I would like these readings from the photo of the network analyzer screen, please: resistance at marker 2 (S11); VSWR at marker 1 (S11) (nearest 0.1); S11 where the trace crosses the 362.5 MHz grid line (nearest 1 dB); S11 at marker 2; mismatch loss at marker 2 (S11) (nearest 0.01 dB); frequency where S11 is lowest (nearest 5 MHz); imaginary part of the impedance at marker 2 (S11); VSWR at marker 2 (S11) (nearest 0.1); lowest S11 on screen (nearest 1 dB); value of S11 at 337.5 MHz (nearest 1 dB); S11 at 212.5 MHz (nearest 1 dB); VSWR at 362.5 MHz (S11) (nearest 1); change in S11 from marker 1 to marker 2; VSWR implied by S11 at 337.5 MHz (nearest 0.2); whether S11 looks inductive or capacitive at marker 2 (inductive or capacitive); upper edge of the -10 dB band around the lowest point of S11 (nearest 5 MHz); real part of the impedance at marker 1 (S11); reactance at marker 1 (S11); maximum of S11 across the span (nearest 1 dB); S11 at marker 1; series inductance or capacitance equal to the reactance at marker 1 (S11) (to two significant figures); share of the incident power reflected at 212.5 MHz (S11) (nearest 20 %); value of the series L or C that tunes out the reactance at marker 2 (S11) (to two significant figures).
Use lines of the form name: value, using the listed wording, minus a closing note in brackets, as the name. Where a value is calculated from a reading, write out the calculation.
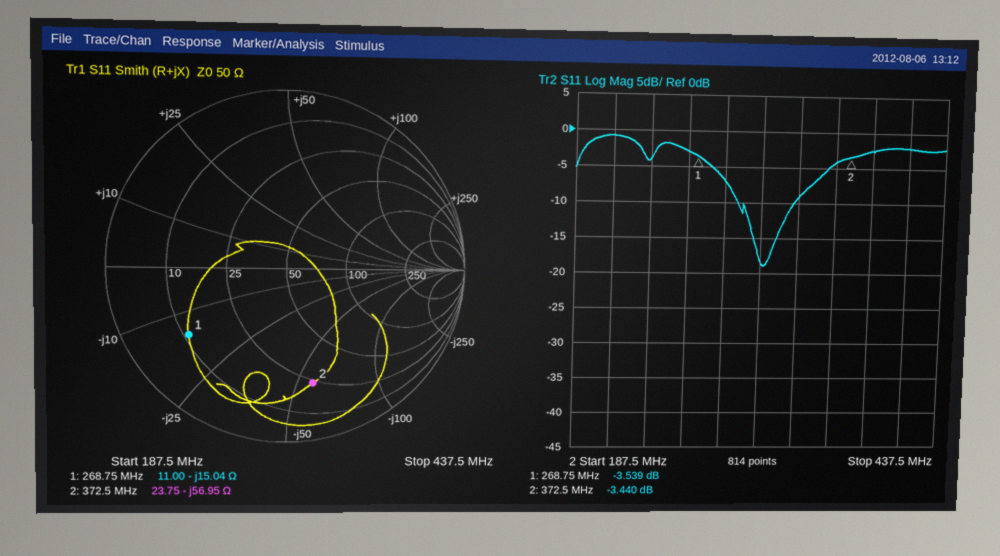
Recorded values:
resistance at marker 2: 23.75 Ω
VSWR at marker 1 (S11): 5.0
S11 where the trace crosses the 362.5 MHz grid line: -4 dB
S11 at marker 2: -3.440 dB
mismatch loss at marker 2 (S11): −10 log10(1 − 10^(-3.44/10)) ≈ 2.62 dB
frequency where S11 is lowest: 315 MHz
imaginary part of the impedance at marker 2: -56.95 Ω
VSWR at marker 2 (S11): 5.1
lowest S11 on screen: -19 dB
value of S11 at 337.5 MHz: -9 dB
S11 at 212.5 MHz: -1 dB
VSWR at 362.5 MHz (S11): |Γ| = 10^(-4/20) = 0.6310; VSWR = (1 + 0.6310)/(1 − 0.6310) ≈ 4
change in S11 from marker 1 to marker 2: -3.44 − (-3.539) = 0.099 dB
VSWR implied by S11 at 337.5 MHz: |Γ| = 10^(-9/20) = 0.3548; VSWR = (1 + 0.3548)/(1 − 0.3548) ≈ 2.10, so 2.0 to the nearest 0.2
whether S11 looks inductive or capacitive at marker 2: capacitive
upper edge of the -10 dB band around the lowest point of S11: 335 MHz
real part of the impedance at marker 1: 11.00 Ω
reactance at marker 1: -15.04 Ω
maximum of S11 across the span: -1 dB
S11 at marker 1: -3.539 dB
series inductance or capacitance equal to the reactance at marker 1 (S11): C = 1/(2π × 268.75 MHz × 15.04 Ω) ≈ 39 pF
share of the incident power reflected at 212.5 MHz (S11): 10^(-1/10) ≈ 79.4 %, so 80 % to the nearest 20 %
value of the series L or C that tunes out the reactance at marker 2 (S11): L = 56.95 Ω/(2π × 372.5 MHz) ≈ 24 nH
